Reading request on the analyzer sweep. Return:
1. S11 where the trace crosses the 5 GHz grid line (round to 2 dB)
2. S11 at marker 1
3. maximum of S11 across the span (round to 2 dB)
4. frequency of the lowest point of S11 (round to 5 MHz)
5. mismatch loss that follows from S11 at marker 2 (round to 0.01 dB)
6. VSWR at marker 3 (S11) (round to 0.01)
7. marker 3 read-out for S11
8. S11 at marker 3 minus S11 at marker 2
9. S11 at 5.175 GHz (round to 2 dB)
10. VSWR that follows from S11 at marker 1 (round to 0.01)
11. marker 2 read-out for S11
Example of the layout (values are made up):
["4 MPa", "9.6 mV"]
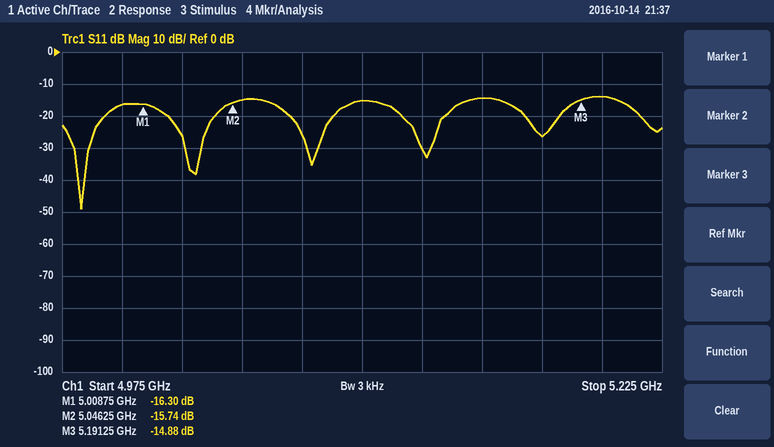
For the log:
["-16 dB", "-16.30 dB", "-14 dB", "4.985 GHz", "0.12 dB", "1.44", "-14.88 dB", "0.86 dB", "-26 dB", "1.36", "-15.74 dB"]
